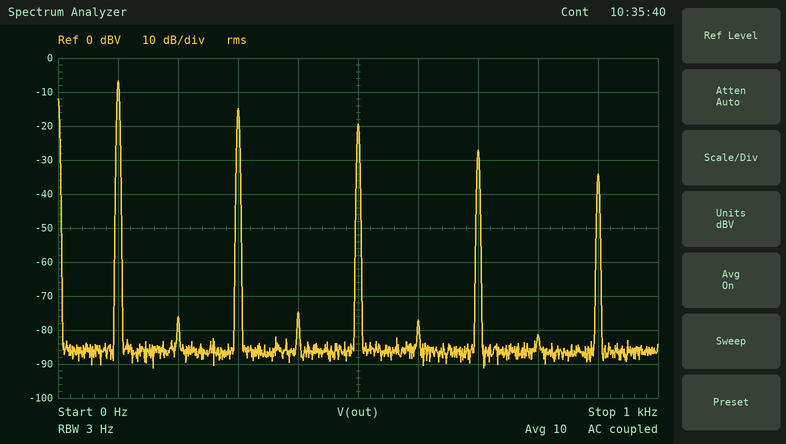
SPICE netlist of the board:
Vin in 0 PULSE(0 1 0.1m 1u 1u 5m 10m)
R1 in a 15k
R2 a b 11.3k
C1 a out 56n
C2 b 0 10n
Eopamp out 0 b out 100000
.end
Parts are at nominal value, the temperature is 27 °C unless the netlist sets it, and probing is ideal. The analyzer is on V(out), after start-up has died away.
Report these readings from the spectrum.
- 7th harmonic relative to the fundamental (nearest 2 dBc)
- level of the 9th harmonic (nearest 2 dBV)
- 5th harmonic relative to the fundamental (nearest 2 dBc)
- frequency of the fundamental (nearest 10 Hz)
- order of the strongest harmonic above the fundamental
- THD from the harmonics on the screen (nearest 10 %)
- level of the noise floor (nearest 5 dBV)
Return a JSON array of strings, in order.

["-20 dBc", "-34 dBV", "-12 dBc", "100 Hz", "3", "50 %", "-85 dBV"]
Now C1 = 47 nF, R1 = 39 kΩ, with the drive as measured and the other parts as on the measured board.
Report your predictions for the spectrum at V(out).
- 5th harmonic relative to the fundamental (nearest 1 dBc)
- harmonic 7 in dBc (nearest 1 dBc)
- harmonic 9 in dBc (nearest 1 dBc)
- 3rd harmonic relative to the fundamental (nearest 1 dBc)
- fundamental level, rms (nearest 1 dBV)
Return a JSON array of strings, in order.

["-20 dBc", "-29 dBc", "-35 dBc", "-10 dBc", "-7 dBV"]
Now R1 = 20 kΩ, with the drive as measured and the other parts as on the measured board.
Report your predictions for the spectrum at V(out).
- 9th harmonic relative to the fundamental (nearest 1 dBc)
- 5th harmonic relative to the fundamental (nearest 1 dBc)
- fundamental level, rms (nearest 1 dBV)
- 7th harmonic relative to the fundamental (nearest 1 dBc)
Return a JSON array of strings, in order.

["-30 dBc", "-14 dBc", "-7 dBV", "-23 dBc"]
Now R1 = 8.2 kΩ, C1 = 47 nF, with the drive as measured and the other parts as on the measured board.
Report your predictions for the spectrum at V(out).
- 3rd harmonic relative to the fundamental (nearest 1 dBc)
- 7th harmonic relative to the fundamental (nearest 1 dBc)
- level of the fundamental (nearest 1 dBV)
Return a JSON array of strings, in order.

["-9 dBc", "-16 dBc", "-7 dBV"]
